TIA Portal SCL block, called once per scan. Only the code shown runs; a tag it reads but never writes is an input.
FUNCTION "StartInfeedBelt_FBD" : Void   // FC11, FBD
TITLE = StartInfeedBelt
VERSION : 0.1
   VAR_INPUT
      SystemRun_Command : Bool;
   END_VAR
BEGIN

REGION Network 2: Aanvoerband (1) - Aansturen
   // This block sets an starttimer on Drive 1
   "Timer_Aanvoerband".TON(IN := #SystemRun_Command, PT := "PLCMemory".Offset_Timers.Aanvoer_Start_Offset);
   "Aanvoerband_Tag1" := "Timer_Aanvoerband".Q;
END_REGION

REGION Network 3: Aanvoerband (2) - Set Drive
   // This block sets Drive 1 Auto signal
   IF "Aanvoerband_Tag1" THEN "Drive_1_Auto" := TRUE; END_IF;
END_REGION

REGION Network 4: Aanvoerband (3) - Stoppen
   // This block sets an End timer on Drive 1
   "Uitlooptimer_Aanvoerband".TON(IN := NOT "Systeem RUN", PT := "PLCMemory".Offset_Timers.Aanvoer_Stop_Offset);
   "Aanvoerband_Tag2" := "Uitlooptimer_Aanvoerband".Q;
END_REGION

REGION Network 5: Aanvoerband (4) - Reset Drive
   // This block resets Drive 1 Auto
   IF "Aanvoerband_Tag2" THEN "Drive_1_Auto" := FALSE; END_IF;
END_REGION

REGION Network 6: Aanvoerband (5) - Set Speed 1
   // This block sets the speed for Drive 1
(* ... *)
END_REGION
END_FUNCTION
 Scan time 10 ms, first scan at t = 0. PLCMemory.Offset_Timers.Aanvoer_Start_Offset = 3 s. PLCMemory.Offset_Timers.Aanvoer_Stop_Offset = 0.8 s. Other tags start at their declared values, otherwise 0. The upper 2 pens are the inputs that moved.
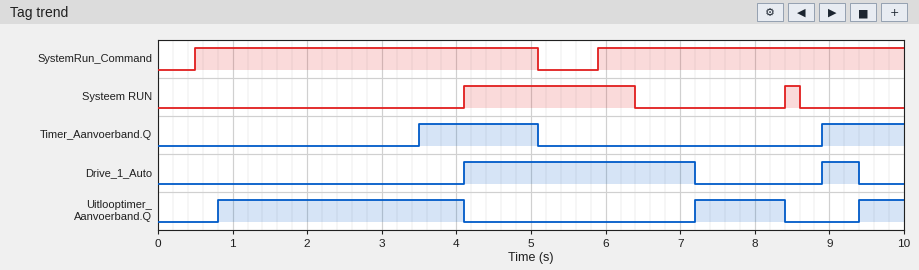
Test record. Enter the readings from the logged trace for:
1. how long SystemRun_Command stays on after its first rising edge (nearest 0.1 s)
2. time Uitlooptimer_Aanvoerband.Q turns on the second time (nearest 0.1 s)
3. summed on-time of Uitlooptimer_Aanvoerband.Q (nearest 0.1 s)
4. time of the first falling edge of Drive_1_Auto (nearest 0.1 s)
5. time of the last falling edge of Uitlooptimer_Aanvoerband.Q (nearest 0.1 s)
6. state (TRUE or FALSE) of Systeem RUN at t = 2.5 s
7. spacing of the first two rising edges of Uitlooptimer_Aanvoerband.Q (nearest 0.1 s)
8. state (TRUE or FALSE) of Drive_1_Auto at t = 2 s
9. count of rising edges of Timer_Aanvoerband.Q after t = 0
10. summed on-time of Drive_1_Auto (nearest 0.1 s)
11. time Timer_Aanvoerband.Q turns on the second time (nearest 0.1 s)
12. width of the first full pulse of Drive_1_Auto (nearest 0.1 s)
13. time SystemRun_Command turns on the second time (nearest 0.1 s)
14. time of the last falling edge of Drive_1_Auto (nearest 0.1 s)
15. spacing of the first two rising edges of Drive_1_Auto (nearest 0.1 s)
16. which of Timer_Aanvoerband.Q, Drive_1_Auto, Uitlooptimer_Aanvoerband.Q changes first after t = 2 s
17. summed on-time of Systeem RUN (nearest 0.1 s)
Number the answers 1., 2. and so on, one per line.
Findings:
1. 4.6 s
2. 7.2 s
3. 5.1 s
4. 7.2 s
5. 8.4 s
6. FALSE
7. 6.4 s
8. FALSE
9. 2
10. 3.6 s
11. 8.9 s
12. 3.1 s
13. 5.9 s
14. 9.4 s
15. 4.8 s
16. Timer_Aanvoerband.Q
17. 2.5 s
